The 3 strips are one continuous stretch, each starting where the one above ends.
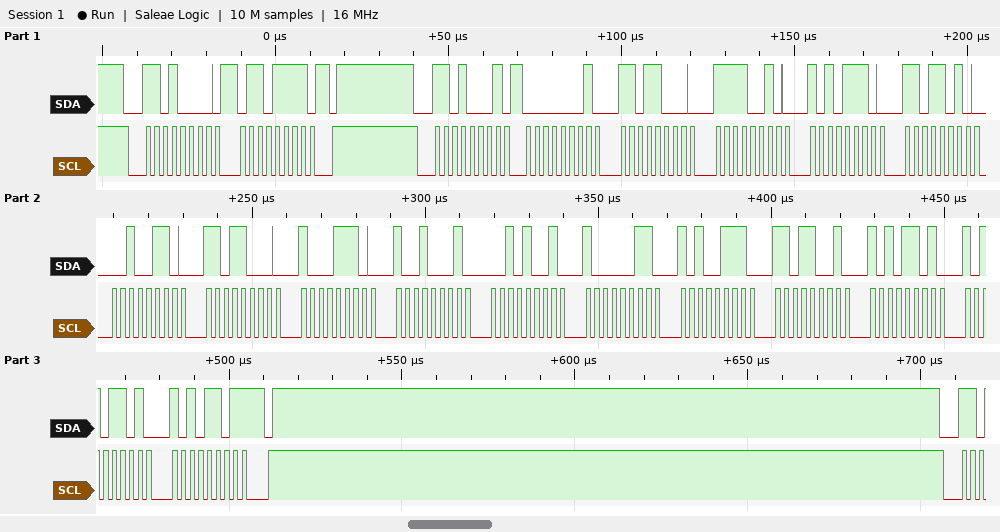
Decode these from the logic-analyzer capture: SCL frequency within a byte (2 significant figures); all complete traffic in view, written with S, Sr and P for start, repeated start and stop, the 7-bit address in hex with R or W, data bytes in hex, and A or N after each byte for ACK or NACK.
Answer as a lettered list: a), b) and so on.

a) 400 kHz
b) S 68W A 6F A P S 68R A 01 A D8 A F2 A AE A DA A 26 A D8 A 8E A 91 A 29 A 83 A A7 A D9 A AD A AD A AD N P
